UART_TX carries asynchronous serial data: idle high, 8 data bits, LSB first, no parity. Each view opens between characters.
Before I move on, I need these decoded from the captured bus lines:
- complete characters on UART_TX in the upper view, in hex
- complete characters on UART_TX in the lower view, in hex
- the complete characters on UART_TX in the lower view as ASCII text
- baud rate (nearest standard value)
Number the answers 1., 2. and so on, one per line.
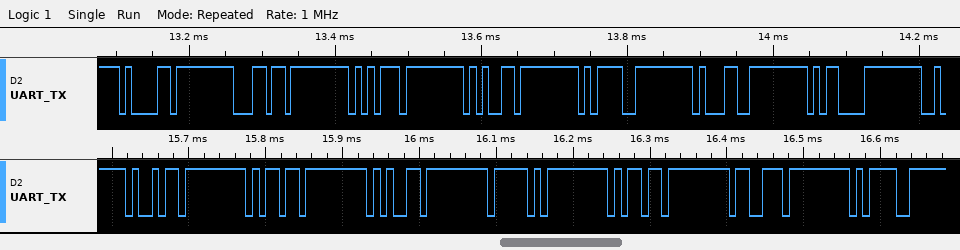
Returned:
1. 61, 6C, 75, 65, 3D, 31, 0D
2. 69, 6D, 65, 5F, 6D, 73, 3D
3. "ime_ms="
4. 115200 baud
